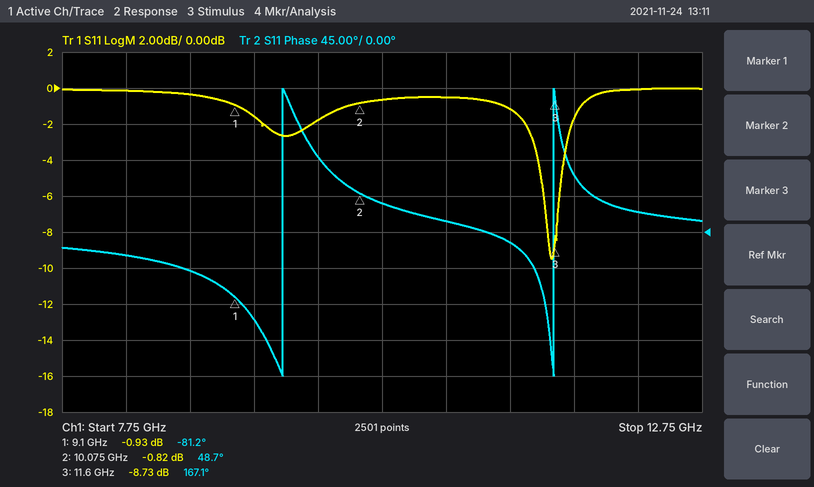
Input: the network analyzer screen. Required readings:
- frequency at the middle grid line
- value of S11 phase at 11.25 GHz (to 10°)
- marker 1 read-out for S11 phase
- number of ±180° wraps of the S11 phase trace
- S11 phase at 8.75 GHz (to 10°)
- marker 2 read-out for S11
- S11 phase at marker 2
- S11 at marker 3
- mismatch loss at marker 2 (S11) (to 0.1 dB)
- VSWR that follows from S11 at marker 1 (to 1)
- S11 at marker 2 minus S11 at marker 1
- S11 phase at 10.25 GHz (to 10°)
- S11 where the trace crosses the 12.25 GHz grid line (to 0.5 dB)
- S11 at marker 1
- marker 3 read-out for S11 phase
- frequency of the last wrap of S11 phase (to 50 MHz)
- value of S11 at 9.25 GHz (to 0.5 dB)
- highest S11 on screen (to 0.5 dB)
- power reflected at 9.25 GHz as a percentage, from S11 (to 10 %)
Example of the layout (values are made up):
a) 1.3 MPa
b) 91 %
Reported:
a) 10.25 GHz
b) -10°
c) -81.2°
d) 2
e) -50°
f) -0.82 dB
g) 48.7°
h) -8.73 dB
i) 7.6 dB
j) 19
k) 0.11 dB
l) 40°
m) 0.0 dB
n) -0.93 dB
o) 167.1°
p) 11.60 GHz
q) -1.5 dB
r) 0.0 dB
s) 70 %
